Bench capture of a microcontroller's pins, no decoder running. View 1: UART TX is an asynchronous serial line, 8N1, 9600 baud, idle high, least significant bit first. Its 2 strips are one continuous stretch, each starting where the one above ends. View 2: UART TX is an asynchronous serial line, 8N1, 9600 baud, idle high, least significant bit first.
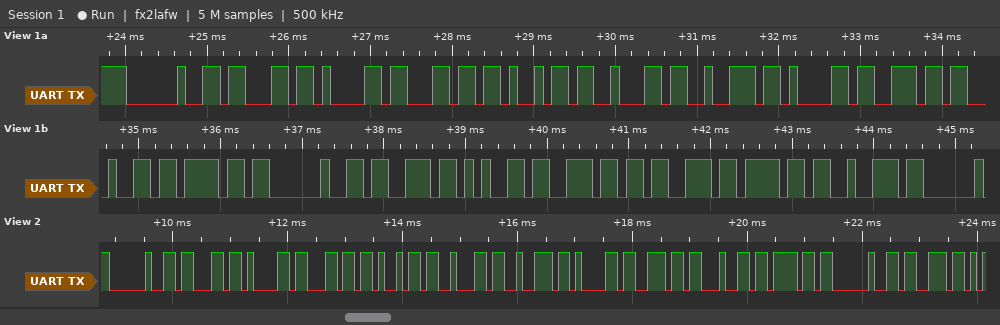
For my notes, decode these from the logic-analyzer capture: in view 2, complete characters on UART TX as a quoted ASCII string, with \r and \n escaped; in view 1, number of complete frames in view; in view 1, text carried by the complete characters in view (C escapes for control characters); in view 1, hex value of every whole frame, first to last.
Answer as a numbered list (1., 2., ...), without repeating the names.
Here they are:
1. " calibrando s"
2. 18
3. " calibrando sensor"
4. 20 63 61 6C 69 62 72 61 6E 64 6F 20 73 65 6E 73 6F 72
